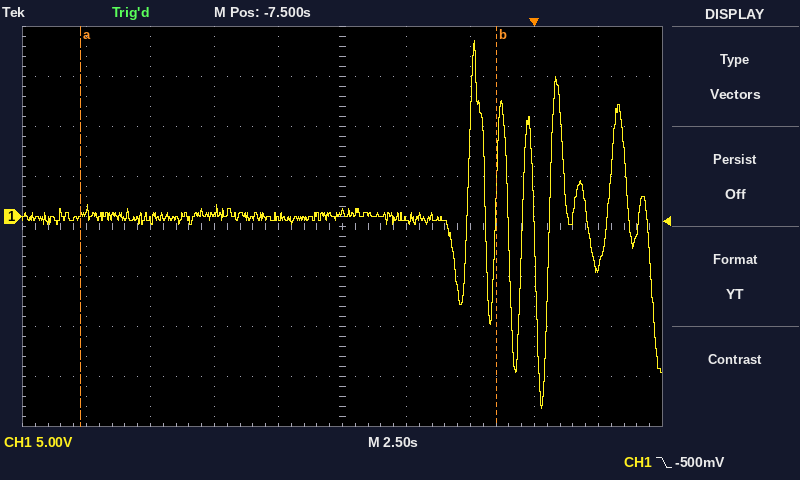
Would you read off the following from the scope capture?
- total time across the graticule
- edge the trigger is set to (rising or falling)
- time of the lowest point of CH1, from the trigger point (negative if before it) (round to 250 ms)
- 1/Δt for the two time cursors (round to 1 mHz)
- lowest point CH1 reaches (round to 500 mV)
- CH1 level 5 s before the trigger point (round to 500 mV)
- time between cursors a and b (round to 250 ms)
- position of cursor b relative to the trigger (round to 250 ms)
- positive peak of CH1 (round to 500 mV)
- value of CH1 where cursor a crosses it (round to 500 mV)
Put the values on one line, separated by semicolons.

25 s; falling; +250 ms; 62 mHz; -19.0 V; -500 mV; 16.25 s; -1.50 s; 17.5 V; 0.0 V
